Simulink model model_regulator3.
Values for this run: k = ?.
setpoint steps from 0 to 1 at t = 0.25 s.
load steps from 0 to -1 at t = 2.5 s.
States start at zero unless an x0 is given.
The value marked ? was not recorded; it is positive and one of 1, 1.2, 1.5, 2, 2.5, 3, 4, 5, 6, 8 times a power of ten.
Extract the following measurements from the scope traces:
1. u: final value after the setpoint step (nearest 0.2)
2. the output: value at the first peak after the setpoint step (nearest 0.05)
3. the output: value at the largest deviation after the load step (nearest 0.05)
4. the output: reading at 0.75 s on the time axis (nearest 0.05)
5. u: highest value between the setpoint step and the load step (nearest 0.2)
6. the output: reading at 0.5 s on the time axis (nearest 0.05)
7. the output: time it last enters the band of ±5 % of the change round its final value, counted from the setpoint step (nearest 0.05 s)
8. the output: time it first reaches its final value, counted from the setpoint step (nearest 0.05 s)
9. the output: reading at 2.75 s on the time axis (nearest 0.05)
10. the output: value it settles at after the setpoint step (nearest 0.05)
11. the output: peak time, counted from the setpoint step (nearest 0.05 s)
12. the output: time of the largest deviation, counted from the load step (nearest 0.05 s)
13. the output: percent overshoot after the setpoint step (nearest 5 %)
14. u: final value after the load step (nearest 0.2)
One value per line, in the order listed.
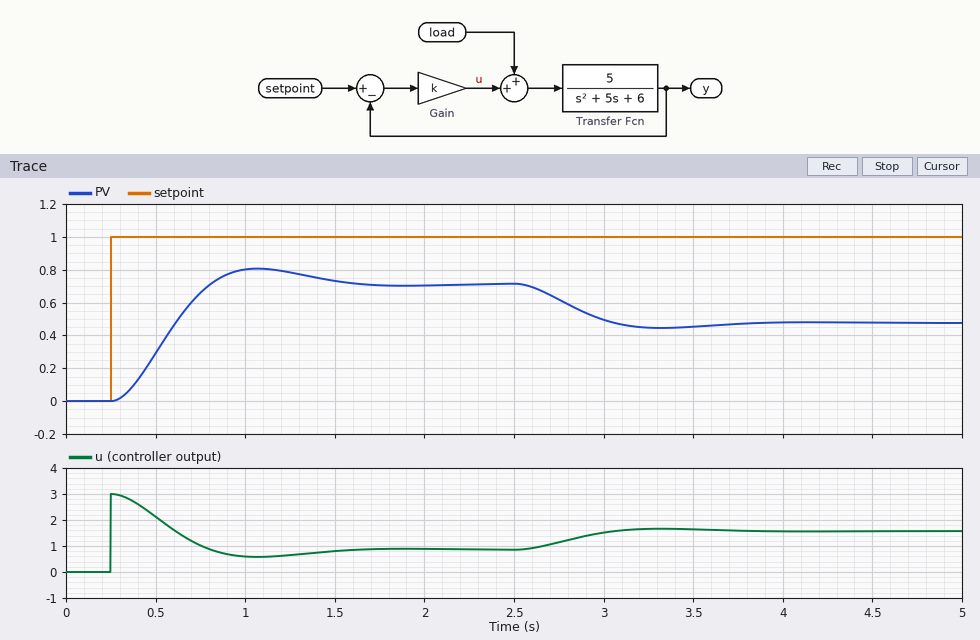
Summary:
0.8
0.80
0.45
0.65
3.0
0.30
1.15 s
0.55 s
0.60
0.70
0.80 s
0.80 s
15 %
1.6
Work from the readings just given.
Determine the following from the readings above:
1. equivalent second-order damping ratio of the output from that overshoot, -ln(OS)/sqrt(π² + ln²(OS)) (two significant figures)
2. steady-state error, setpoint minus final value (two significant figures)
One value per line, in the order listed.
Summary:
0.52
0.30
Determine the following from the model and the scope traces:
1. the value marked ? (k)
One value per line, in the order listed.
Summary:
3
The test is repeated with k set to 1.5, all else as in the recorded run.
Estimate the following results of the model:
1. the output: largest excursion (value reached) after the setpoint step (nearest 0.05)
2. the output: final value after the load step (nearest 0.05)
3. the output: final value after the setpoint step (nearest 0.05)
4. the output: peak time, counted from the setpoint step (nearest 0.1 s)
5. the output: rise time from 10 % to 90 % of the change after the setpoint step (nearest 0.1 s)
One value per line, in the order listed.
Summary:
0.60
0.20
0.55
1.2 s
0.6 s
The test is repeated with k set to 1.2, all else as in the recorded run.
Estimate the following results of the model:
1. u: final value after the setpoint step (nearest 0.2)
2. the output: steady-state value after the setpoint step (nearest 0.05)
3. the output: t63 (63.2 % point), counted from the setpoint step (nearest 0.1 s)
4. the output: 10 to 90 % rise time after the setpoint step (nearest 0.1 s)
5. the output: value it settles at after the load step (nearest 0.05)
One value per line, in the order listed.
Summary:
0.6
0.50
0.5 s
0.6 s
0.10
